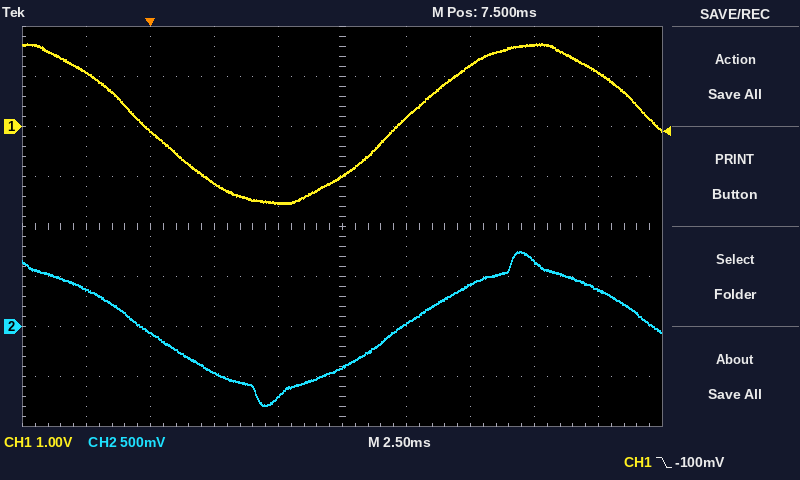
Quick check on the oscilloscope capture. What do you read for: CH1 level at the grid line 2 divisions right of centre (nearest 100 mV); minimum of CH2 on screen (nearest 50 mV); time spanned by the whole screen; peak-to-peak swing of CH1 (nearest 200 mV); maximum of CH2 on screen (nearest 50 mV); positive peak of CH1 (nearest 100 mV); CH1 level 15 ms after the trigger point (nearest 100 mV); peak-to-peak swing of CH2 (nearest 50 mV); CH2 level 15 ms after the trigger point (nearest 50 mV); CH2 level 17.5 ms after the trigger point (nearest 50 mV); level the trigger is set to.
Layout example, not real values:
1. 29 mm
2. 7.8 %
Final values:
1. 1.2 V
2. -800 mV
3. 25 ms
4. 3.2 V
5. 750 mV
6. 1.7 V
7. 1.6 V
8. 1.55 V
9. 650 mV
10. 350 mV
11. -100 mV
